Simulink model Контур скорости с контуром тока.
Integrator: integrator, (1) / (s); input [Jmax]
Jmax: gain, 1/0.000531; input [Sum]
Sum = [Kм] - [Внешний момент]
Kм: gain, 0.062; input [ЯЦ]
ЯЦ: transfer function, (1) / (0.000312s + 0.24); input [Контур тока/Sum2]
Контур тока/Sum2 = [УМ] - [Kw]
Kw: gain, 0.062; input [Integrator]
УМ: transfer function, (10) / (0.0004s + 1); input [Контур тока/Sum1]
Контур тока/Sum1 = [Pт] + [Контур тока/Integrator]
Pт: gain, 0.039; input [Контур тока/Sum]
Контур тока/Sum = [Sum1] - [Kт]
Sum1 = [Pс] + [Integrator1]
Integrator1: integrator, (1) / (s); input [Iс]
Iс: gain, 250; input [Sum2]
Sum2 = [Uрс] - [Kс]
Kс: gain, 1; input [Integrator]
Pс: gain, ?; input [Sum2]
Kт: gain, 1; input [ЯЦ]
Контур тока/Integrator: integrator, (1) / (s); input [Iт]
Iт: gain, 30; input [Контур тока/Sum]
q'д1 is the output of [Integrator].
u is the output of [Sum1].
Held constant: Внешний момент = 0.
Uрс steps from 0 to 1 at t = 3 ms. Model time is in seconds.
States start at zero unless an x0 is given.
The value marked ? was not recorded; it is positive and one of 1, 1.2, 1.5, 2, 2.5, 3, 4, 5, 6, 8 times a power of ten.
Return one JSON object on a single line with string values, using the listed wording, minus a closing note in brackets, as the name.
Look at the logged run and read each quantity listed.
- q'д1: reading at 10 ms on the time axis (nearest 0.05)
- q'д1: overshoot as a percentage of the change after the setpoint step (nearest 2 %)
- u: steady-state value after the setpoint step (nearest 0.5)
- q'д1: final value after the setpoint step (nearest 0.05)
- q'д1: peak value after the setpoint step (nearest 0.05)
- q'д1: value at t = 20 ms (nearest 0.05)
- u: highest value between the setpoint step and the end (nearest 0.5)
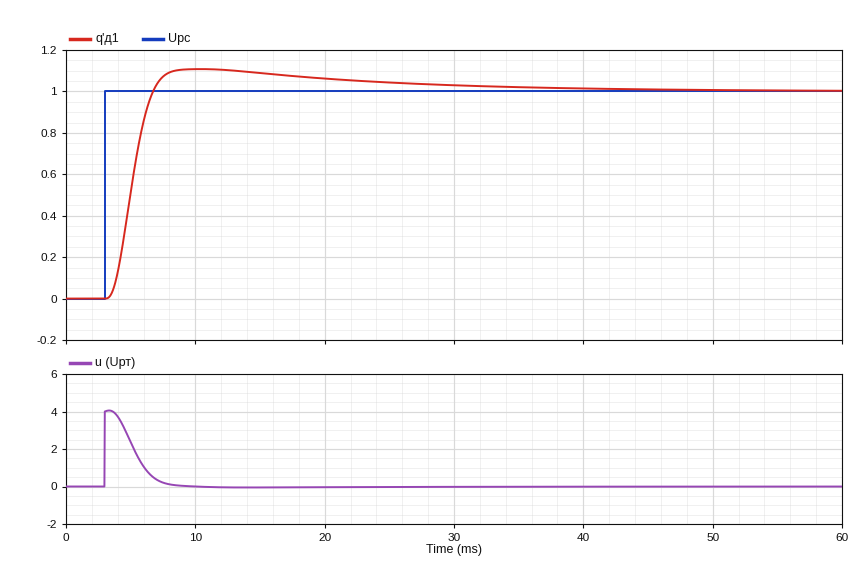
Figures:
{"q'д1: reading at 10 ms on the time axis": "1.10", "q'д1: overshoot as a percentage of the change after the setpoint step": "10 %", "u: steady-state value after the setpoint step": "0.0", "q'д1: final value after the setpoint step": "1.00", "q'д1: peak value after the setpoint step": "1.10", "q'д1: value at t = 20 ms": "1.05", "u: highest value between the setpoint step and the end": "4.0"}
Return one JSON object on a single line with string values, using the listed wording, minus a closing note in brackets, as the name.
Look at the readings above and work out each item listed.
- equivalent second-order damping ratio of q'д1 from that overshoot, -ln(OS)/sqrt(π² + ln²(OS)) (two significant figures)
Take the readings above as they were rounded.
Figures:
{"equivalent second-order damping ratio of q'д1 from that overshoot, -ln(OS)/sqrt(π² + ln²(OS))": "0.59"}
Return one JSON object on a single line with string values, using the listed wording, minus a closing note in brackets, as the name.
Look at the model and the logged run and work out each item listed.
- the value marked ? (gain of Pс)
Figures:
{"the value marked ?": "4"}
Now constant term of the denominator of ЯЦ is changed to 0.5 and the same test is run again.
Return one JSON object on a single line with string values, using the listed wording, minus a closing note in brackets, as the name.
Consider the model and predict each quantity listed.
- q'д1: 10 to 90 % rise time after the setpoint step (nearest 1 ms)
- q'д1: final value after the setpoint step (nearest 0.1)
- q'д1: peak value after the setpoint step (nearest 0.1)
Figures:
{"q'д1: 10 to 90 % rise time after the setpoint step": "3 ms", "q'д1: final value after the setpoint step": "1.0", "q'д1: peak value after the setpoint step": "1.2"}
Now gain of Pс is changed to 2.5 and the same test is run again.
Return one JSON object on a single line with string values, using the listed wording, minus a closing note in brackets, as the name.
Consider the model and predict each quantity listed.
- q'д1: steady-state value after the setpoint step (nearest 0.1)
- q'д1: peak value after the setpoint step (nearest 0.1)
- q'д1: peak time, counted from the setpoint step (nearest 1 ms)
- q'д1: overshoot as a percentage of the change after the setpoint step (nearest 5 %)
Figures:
{"q'д1: steady-state value after the setpoint step": "1.0", "q'д1: peak value after the setpoint step": "1.2", "q'д1: peak time, counted from the setpoint step": "11 ms", "q'д1: overshoot as a percentage of the change after the setpoint step": "20 %"}
